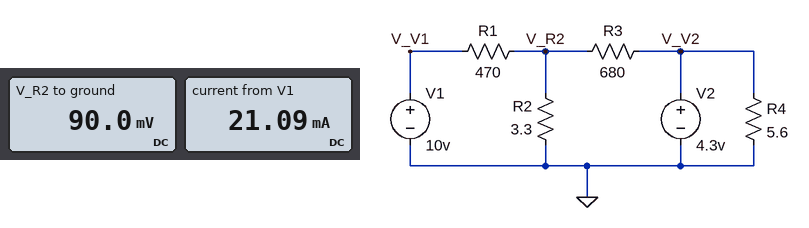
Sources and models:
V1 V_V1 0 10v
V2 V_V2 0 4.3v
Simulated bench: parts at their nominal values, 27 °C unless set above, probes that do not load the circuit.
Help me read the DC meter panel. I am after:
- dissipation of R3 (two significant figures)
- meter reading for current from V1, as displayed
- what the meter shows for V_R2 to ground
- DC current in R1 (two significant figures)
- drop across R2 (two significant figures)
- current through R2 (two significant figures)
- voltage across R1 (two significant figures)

26 mW
21.09 mA
90.0 mV
21 mA
90 mV
27 mA
9.9 V
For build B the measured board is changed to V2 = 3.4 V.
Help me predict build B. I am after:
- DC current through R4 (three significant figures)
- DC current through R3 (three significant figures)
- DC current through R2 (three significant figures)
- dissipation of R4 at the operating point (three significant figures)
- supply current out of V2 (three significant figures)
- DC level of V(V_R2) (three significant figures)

607 mA
4.87 mA
26.0 mA
2.06 W
612 mA
85.7 mV
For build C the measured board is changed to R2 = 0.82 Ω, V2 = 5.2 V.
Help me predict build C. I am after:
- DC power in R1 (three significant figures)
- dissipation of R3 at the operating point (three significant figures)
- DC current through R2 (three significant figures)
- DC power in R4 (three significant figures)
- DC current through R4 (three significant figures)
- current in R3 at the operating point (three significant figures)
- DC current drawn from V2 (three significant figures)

212 mW
39.4 mW
28.8 mA
4.83 W
929 mA
7.61 mA
936 mA
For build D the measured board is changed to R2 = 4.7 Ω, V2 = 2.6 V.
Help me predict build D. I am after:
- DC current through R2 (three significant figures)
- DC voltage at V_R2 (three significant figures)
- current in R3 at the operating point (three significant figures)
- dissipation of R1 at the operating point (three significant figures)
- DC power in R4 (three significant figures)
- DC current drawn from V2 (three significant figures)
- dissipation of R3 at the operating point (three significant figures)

24.7 mA
116 mV
3.65 mA
208 mW
1.21 W
468 mA
9.07 mW
